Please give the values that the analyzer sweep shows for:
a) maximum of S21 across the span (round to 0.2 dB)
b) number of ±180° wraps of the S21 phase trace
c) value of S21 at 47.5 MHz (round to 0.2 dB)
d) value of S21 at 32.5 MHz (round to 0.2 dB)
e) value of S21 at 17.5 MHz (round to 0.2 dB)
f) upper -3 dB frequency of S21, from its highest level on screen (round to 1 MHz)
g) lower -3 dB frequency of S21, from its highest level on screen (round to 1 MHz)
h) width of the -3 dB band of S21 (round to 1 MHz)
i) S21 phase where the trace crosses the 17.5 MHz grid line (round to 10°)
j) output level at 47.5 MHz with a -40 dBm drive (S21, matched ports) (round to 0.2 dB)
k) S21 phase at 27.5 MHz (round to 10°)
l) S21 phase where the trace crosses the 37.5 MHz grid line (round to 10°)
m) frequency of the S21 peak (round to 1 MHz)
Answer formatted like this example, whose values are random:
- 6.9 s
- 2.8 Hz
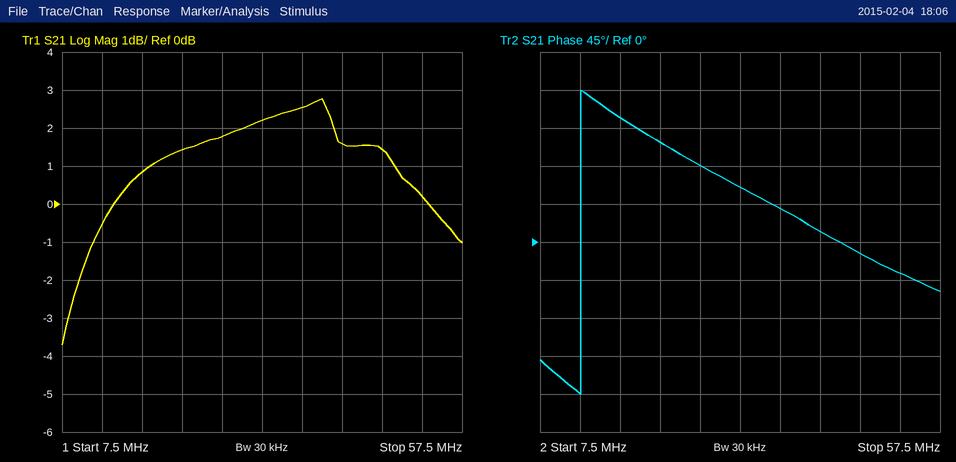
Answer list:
- 2.8 dB
- 1
- 1.4 dB
- 2.2 dB
- 0.8 dB
- 54 MHz
- 13 MHz
- 41 MHz
- 150°
- -38.6 dBm
- 90°
- 40°
- 40 MHz
